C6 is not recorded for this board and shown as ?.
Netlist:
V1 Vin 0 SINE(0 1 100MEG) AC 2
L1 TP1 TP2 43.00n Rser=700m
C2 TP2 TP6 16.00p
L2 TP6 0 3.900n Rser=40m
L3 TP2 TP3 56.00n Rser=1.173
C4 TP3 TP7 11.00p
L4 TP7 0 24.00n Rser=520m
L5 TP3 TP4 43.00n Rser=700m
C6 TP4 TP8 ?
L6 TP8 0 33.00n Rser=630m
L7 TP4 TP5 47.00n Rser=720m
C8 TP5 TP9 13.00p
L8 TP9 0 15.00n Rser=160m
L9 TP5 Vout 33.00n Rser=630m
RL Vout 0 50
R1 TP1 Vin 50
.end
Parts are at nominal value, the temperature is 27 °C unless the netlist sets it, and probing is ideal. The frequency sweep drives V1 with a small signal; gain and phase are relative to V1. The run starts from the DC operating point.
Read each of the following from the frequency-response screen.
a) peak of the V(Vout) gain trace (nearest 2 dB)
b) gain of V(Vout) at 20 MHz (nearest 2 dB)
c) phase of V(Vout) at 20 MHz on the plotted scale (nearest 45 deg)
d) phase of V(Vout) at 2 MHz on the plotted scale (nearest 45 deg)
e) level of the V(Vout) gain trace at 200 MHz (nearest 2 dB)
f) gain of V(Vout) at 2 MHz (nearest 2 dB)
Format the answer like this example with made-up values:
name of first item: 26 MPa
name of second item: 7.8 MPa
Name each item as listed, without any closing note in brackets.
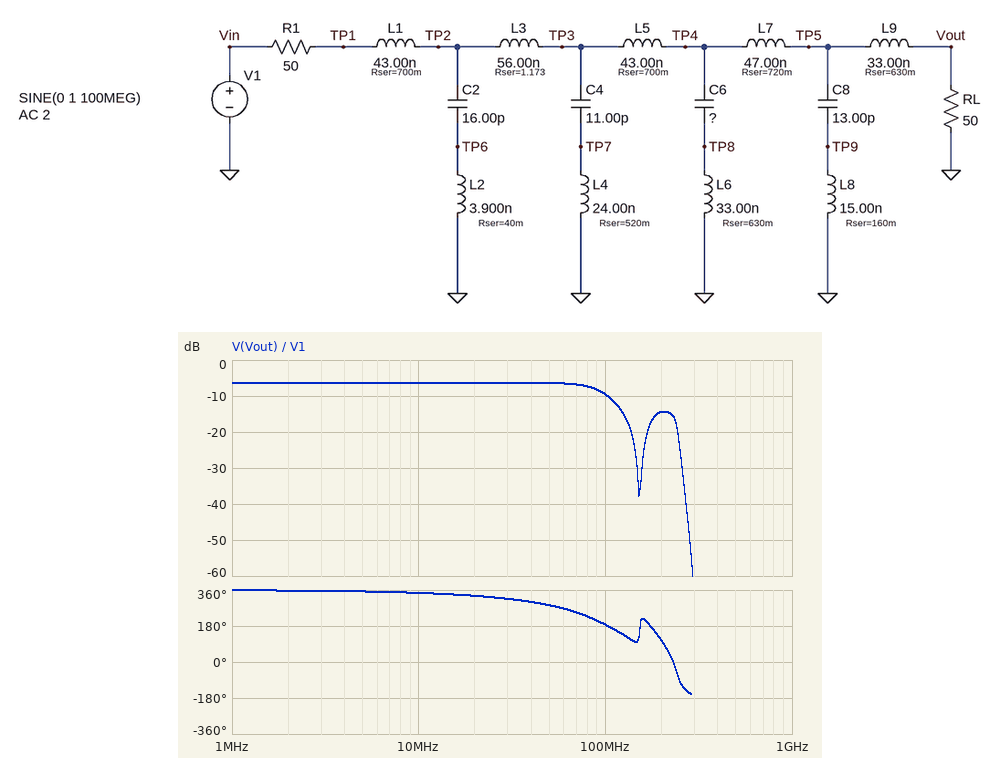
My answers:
peak of the V(Vout) gain trace: -6 dB
gain of V(Vout) at 20 MHz: -6 dB
phase of V(Vout) at 20 MHz on the plotted scale: 315 deg
phase of V(Vout) at 2 MHz on the plotted scale: 360 deg
level of the V(Vout) gain trace at 200 MHz: -14 dB
gain of V(Vout) at 2 MHz: -6 dB
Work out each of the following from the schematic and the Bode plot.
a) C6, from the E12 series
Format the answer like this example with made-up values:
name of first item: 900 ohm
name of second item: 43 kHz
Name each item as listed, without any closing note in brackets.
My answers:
C6, from the E12 series: 33 pF
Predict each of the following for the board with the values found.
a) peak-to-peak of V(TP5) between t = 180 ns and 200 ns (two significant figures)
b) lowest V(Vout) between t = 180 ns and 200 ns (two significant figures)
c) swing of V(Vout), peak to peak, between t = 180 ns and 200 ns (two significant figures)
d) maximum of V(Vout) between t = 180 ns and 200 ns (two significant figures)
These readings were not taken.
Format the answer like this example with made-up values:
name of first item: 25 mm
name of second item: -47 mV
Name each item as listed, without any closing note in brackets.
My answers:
peak-to-peak of V(TP5) between t = 180 ns and 200 ns: 730 mV
lowest V(Vout) between t = 180 ns and 200 ns: -330 mV
swing of V(Vout), peak to peak, between t = 180 ns and 200 ns: 670 mV
maximum of V(Vout) between t = 180 ns and 200 ns: 330 mV
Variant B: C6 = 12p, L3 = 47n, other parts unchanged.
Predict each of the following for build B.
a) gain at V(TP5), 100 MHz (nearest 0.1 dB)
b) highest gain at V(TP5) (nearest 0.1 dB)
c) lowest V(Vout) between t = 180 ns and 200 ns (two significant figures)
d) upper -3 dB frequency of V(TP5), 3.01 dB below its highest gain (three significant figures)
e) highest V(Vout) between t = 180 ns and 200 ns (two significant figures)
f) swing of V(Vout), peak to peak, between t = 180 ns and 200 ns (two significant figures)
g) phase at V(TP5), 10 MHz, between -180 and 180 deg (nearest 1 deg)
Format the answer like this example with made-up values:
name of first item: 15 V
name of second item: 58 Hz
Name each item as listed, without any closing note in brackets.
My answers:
gain at V(TP5), 100 MHz: -5.6 dB
highest gain at V(TP5): -4.6 dB
lowest V(Vout) between t = 180 ns and 200 ns: -480 mV
upper -3 dB frequency of V(TP5), 3.01 dB below its highest gain: 219 MHz
highest V(Vout) between t = 180 ns and 200 ns: 480 mV
swing of V(Vout), peak to peak, between t = 180 ns and 200 ns: 960 mV
phase at V(TP5), 10 MHz, between -180 and 180 deg: -10 deg
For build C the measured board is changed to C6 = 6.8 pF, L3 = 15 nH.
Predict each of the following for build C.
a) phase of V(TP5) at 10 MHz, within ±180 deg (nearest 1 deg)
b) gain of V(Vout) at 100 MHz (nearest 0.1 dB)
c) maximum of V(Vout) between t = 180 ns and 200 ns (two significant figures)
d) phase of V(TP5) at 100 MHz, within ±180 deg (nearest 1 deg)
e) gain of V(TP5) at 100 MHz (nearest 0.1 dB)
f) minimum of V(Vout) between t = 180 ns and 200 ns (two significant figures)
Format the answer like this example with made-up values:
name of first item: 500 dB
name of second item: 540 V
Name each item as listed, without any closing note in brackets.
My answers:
phase of V(TP5) at 10 MHz, within ±180 deg: -8 deg
gain of V(Vout) at 100 MHz: -6.4 dB
maximum of V(Vout) between t = 180 ns and 200 ns: 480 mV
phase of V(TP5) at 100 MHz, within ±180 deg: -89 deg
gain of V(TP5) at 100 MHz: -5.6 dB
minimum of V(Vout) between t = 180 ns and 200 ns: -480 mV
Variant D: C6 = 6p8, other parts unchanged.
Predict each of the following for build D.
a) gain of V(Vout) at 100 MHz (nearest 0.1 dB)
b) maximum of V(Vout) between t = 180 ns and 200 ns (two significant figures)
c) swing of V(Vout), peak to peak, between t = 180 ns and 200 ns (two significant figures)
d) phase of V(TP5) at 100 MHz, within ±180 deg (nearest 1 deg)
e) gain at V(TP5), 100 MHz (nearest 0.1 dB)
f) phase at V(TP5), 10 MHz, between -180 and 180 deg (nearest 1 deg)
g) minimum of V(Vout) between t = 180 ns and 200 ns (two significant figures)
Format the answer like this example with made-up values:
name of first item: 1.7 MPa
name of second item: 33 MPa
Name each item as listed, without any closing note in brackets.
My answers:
gain of V(Vout) at 100 MHz: -6.4 dB
maximum of V(Vout) between t = 180 ns and 200 ns: 480 mV
swing of V(Vout), peak to peak, between t = 180 ns and 200 ns: 960 mV
phase of V(TP5) at 100 MHz, within ±180 deg: -99 deg
gain at V(TP5), 100 MHz: -5.6 dB
phase at V(TP5), 10 MHz, between -180 and 180 deg: -10 deg
minimum of V(Vout) between t = 180 ns and 200 ns: -480 mV
